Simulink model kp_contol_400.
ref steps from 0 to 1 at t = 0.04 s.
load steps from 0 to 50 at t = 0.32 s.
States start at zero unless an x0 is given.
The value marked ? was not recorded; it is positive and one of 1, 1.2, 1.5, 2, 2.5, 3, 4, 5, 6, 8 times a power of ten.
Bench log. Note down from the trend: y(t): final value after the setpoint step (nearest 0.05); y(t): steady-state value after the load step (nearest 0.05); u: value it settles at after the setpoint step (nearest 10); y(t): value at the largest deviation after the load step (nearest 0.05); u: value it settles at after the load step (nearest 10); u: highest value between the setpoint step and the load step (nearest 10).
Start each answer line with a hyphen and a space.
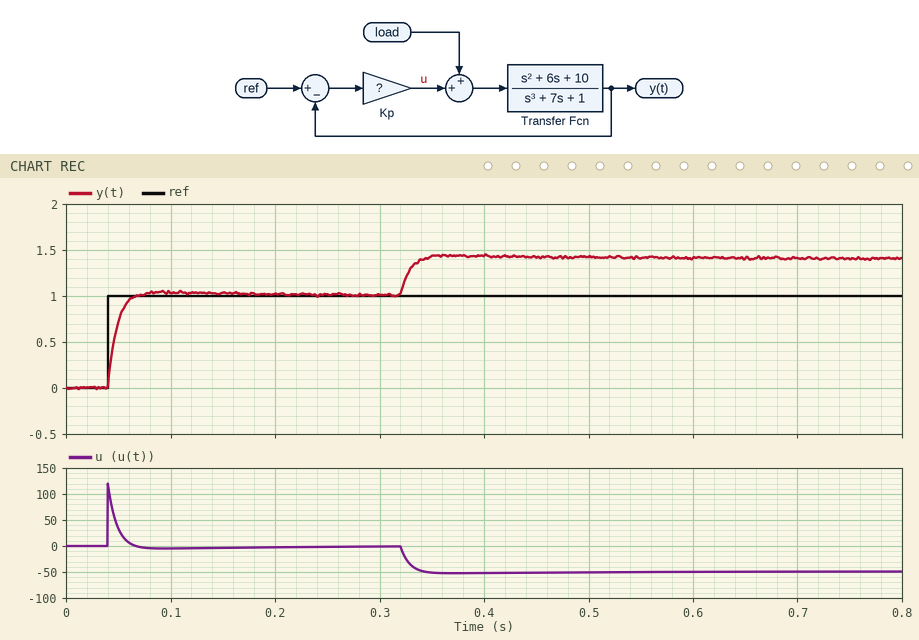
- 1.00
- 1.40
- 0
- 1.45
- -50
- 120
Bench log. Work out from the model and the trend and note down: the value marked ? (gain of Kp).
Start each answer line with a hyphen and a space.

- 120
